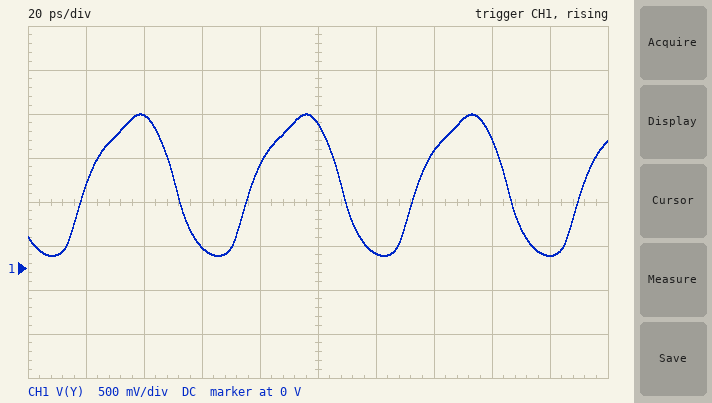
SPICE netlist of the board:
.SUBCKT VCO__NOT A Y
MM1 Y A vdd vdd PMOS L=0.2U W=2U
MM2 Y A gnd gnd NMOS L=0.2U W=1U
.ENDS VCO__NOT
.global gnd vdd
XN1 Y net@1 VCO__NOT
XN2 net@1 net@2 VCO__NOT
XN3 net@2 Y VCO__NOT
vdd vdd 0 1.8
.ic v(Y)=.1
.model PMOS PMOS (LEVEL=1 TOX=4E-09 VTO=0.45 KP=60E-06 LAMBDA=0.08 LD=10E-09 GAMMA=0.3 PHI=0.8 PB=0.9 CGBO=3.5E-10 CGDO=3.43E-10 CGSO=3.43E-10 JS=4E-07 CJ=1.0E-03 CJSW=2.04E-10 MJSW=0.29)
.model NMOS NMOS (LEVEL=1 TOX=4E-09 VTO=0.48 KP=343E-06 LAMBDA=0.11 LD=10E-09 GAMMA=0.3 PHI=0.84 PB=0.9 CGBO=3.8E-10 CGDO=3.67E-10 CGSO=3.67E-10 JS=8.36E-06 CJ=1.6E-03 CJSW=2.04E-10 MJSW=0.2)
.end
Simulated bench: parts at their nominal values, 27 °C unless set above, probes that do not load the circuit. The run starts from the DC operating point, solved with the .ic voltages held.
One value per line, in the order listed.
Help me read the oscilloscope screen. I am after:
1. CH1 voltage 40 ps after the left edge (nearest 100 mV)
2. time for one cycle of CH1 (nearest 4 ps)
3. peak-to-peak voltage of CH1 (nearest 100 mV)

1.7 V
56 ps
1.6 V
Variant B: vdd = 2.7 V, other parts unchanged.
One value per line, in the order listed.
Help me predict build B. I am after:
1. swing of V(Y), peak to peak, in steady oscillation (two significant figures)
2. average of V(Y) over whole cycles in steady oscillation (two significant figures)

2.3 V
1.3 V
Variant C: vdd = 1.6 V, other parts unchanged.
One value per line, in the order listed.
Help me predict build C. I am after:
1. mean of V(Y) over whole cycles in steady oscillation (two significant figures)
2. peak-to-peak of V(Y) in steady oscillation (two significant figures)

880 mV
1.4 V
